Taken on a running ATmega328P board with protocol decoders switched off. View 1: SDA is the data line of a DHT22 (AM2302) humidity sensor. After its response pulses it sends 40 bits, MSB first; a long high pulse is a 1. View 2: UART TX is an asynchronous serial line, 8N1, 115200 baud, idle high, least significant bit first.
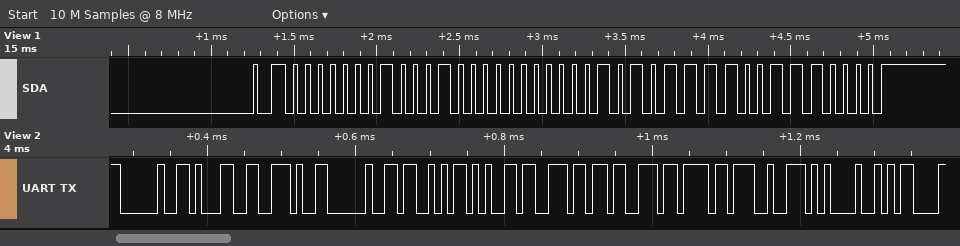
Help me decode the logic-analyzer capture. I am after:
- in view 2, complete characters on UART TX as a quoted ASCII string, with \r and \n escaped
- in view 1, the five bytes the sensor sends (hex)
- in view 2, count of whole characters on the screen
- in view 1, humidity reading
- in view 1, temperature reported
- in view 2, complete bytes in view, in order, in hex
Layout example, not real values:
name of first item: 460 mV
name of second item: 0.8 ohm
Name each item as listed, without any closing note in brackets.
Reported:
in view 2, complete characters on UART TX as a quoted ASCII string, with \r and \n escaped: " 1. Sensor!\r"
in view 1, the five bytes the sensor sends: 01 10 01 5E 70
in view 2, count of whole characters on the screen: 12
in view 1, humidity reading: 27.2 %
in view 1, temperature reported: 35.0 °C
in view 2, complete bytes in view, in order, in hex: 20 31 2E 20 53 65 6E 73 6F 72 21 0D
